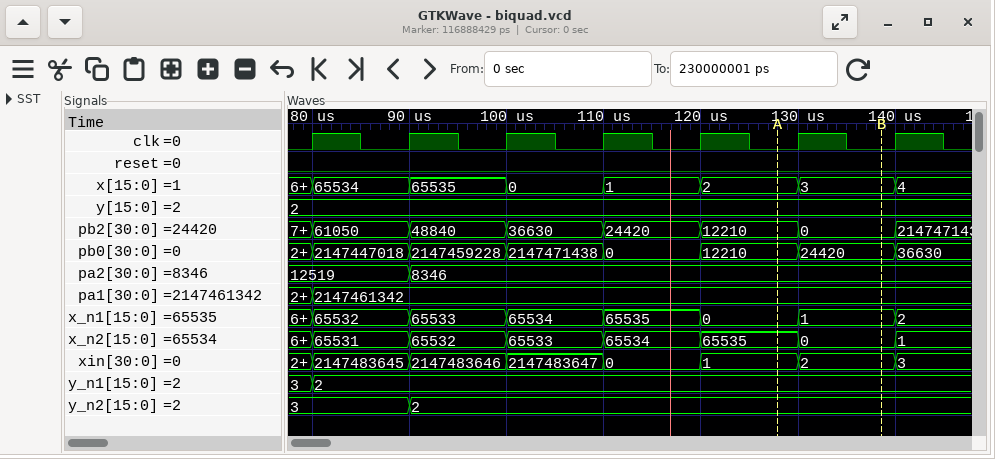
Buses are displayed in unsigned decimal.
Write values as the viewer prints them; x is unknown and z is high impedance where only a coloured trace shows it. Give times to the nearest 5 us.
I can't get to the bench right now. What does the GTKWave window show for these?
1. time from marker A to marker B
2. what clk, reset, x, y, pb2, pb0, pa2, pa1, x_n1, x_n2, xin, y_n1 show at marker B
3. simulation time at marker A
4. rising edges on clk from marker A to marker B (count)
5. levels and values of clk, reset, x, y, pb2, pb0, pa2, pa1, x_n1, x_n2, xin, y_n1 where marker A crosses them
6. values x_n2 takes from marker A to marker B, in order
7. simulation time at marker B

10 us
clk=0, reset=0, x=3, y=2, pb2=0, pb0=24420, pa2=8346, pa1=2147461342, x_n1=1, x_n2=0, xin=2, y_n1=2
130 us
1
clk=0, reset=0, x=2, y=2, pb2=12210, pb0=12210, pa2=8346, pa1=2147461342, x_n1=0, x_n2=65535, xin=1, y_n1=2
65535, 0
140 us
